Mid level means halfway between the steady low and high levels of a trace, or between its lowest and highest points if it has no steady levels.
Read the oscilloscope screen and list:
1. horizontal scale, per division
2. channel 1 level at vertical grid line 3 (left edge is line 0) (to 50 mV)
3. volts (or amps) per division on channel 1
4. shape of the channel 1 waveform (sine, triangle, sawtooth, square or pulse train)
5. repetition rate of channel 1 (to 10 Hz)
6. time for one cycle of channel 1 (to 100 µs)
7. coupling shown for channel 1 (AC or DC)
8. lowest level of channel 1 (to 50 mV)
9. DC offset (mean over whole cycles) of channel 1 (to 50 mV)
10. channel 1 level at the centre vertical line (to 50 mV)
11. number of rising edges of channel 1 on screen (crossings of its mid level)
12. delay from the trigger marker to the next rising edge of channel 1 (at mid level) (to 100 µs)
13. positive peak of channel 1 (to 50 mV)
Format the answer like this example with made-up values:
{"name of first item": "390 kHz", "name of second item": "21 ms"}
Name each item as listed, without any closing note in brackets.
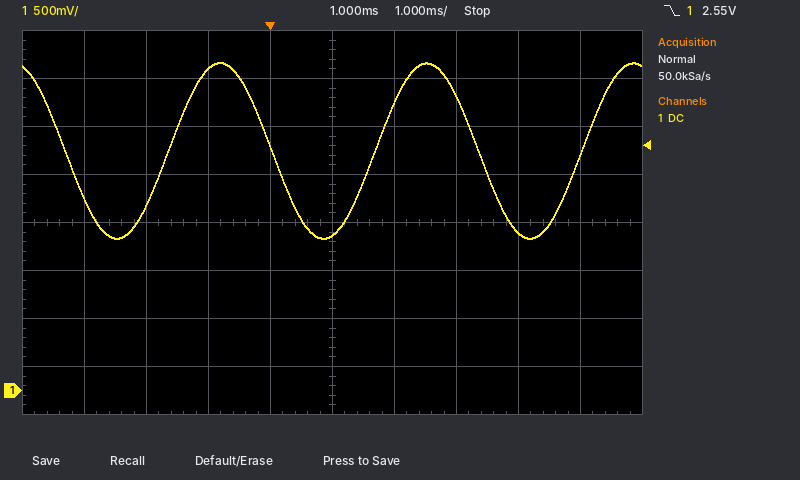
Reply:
{"horizontal scale, per division": "1 ms", "channel 1 level at vertical grid line 3 (left edge is line 0)": "3.35 V", "volts (or amps) per division on channel 1": "500 mV", "shape of the channel 1 waveform": "sine", "repetition rate of channel 1": "300 Hz", "time for one cycle of channel 1": "3.3 ms", "coupling shown for channel 1": "DC", "lowest level of channel 1": "1.60 V", "DC offset (mean over whole cycles) of channel 1": "2.50 V", "channel 1 level at the centre vertical line": "1.60 V", "number of rising edges of channel 1 on screen": "3", "delay from the trigger marker to the next rising edge of channel 1 (at mid level)": "1.7 ms", "positive peak of channel 1": "3.40 V"}
